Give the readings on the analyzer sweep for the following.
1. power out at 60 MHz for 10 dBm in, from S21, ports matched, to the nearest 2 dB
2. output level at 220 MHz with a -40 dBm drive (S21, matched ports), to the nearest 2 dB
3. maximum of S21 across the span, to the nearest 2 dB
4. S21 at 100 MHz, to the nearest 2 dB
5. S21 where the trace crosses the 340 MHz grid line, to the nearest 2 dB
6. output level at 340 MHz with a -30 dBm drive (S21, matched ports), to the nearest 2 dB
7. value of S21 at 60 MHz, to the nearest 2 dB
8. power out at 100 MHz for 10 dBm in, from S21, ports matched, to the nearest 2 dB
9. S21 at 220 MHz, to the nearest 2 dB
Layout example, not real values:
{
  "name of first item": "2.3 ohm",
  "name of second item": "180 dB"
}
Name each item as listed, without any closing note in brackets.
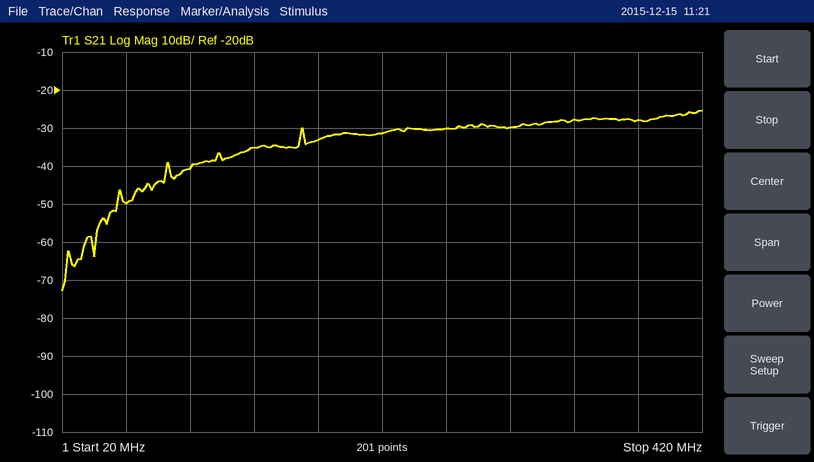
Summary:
{
  "power out at 60 MHz for 10 dBm in, from S21, ports matched, to the nearest 2 dB": "-40 dBm",
  "output level at 220 MHz with a -40 dBm drive (S21, matched ports), to the nearest 2 dB": "-72 dBm",
  "maximum of S21 across the span, to the nearest 2 dB": "-26 dB",
  "S21 at 100 MHz, to the nearest 2 dB": "-40 dB",
  "S21 where the trace crosses the 340 MHz grid line, to the nearest 2 dB": "-28 dB",
  "output level at 340 MHz with a -30 dBm drive (S21, matched ports), to the nearest 2 dB": "-58 dBm",
  "value of S21 at 60 MHz, to the nearest 2 dB": "-50 dB",
  "power out at 100 MHz for 10 dBm in, from S21, ports matched, to the nearest 2 dB": "-30 dBm",
  "S21 at 220 MHz, to the nearest 2 dB": "-32 dB"
}
